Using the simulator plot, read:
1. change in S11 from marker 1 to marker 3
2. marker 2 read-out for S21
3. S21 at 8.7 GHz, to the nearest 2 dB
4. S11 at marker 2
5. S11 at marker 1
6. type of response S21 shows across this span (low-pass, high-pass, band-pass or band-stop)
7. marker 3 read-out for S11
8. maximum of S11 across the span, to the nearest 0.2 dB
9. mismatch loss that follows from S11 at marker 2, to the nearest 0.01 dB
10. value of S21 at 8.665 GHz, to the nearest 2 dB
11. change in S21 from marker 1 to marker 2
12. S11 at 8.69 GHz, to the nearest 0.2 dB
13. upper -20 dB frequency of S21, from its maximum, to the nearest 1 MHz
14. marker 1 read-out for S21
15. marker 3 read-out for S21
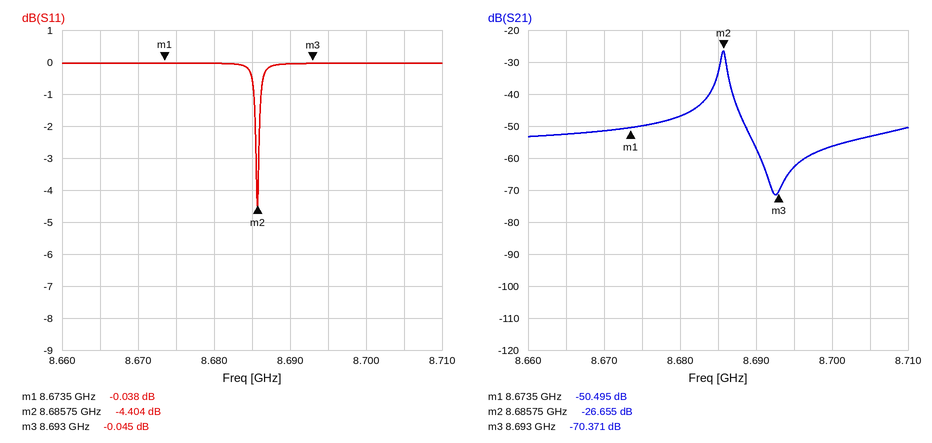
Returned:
-0.007 dB
-26.655 dB
-56 dB
-4.404 dB
-0.038 dB
band-pass
-0.045 dB
0.0 dB
1.96 dB
-52 dB
23.840 dB
0.0 dB
8.688 GHz
-50.495 dB
-70.371 dB
